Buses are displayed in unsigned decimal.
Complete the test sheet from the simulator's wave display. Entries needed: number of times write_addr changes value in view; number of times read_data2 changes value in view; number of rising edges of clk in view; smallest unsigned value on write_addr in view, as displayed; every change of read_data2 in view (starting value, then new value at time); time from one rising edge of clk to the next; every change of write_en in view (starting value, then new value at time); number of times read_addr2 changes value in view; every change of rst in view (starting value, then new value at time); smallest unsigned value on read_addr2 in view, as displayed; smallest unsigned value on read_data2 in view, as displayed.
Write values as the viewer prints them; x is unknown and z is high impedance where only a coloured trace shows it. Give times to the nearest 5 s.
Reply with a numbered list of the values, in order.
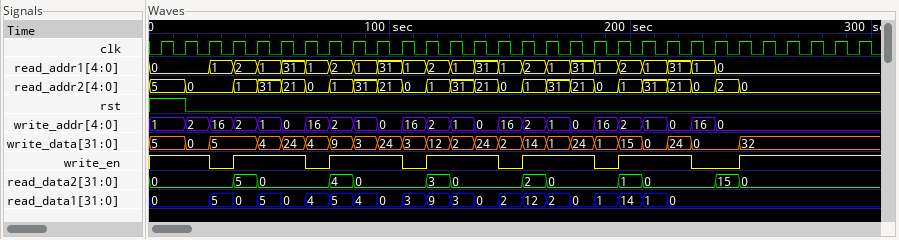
1. 23
2. 12
3. 30
4. 0
5. 0, 5 at 35 s, 0 at 45 s, 4 at 75 s, 0 at 85 s, 3 at 115 s, 0 at 125 s, 2 at 155 s, 0 at 165 s, 1 at 195 s, 0 at 205 s, 15 at 235 s, 0 at 245 s
6. 10 s
7. 1, 0 at 25 s, 1 at 35 s, 0 at 65 s, 1 at 75 s, 0 at 105 s, 1 at 115 s, 0 at 145 s, 1 at 155 s, 0 at 185 s, 1 at 195 s, 0 at 225 s, 1 at 245 s
8. 23
9. 1, 0 at 15 s
10. 0
11. 0
